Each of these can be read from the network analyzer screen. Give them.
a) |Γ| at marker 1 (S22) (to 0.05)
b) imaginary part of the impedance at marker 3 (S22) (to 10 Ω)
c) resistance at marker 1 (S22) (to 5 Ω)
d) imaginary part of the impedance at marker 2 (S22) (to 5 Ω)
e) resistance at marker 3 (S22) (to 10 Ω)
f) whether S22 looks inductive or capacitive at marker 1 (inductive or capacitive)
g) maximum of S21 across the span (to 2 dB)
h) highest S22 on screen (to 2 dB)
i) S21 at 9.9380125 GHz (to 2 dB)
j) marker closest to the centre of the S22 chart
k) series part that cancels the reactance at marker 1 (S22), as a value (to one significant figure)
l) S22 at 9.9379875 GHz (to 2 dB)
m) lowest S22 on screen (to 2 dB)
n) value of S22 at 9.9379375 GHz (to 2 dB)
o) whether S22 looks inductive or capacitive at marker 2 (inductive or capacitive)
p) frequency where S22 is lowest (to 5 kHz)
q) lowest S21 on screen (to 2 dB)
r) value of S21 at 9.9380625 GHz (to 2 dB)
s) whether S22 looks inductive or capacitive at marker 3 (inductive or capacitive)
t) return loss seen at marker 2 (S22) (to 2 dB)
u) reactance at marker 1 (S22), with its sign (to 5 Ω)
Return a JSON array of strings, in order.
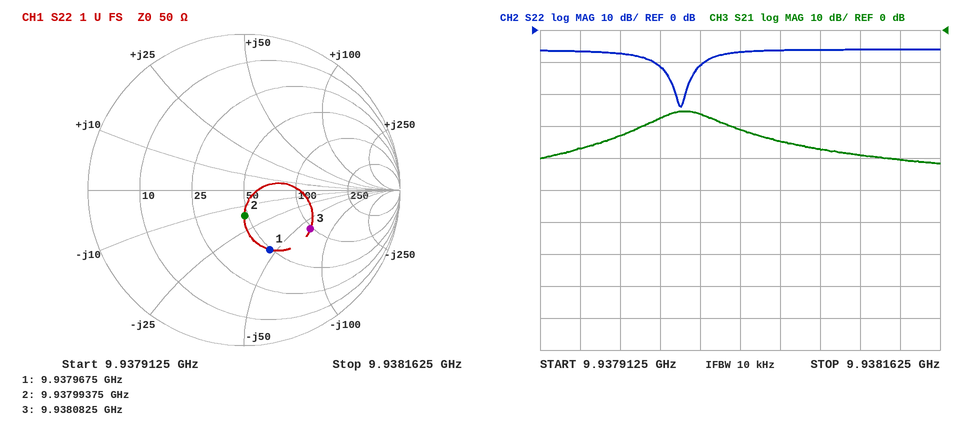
["0.40", "-60 Ω", "50 Ω", "-15 Ω", "100 Ω", "capacitive", "-26 dB", "-6 dB", "-26 dB", "marker 2", "700 pH", "-12 dB", "-24 dB", "-6 dB", "capacitive", "9.938000 GHz", "-42 dB", "-34 dB", "capacitive", "16 dB", "-45 Ω"]
